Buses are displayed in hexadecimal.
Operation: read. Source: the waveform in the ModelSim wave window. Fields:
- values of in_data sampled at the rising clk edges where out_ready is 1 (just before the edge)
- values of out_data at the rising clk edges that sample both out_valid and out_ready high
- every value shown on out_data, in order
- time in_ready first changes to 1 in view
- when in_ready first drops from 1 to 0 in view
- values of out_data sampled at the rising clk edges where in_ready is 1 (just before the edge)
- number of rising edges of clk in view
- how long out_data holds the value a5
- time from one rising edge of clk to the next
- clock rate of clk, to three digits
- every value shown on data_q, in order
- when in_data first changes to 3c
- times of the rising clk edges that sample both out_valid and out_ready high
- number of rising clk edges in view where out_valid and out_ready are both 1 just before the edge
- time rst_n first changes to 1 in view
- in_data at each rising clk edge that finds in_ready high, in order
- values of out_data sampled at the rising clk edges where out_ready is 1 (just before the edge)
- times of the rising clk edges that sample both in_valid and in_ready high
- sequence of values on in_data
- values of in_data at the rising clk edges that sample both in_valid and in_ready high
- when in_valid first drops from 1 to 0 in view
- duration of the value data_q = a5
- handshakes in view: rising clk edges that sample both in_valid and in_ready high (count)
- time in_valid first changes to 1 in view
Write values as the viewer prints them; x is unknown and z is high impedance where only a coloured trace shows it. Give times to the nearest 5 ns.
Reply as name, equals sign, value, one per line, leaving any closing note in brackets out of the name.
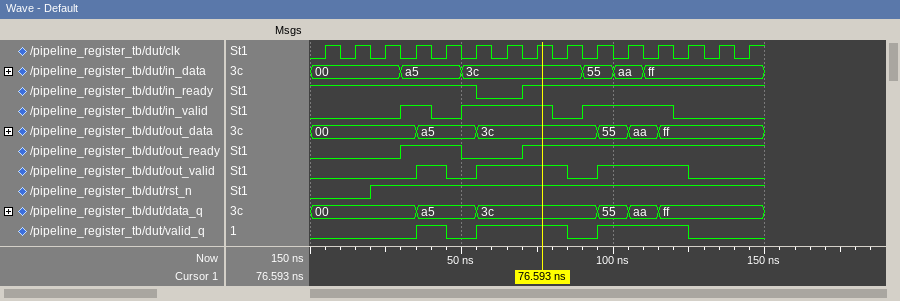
values of in_data sampled at the rising clk edges where out_ready is 1 = a5, a5, 3c, 3c, 55, aa, ff, ff, ff, ff
values of out_data at the rising clk edges that sample both out_valid and out_ready high = a5, 3c, 3c, 55, aa, ff
every value shown on out_data, in order = 00, a5, 3c, 55, aa, ff
time in_ready first changes to 1 in view = 70 ns
when in_ready first drops from 1 to 0 in view = 55 ns
values of out_data sampled at the rising clk edges where in_ready is 1 = 00, 00, 00, 00, a5, a5, 3c, 3c, 3c, 55, aa, ff, ff, ff
number of rising edges of clk in view = 15
how long out_data holds the value a5 = 20 ns
time from one rising edge of clk to the next = 10 ns
clock rate of clk, to three digits = 100 MHz
every value shown on data_q, in order = 00, a5, 3c, 55, aa, ff
when in_data first changes to 3c = 50 ns
times of the rising clk edges that sample both out_valid and out_ready high = 45 ns, 75 ns, 85 ns, 105 ns, 115 ns, 125 ns
number of rising clk edges in view where out_valid and out_ready are both 1 just before the edge = 6
time rst_n first changes to 1 in view = 20 ns
in_data at each rising clk edge that finds in_ready high, in order = 00, 00, 00, a5, a5, 3c, 3c, 3c, 55, aa, ff, ff, ff, ff
values of out_data sampled at the rising clk edges where out_ready is 1 = 00, a5, 3c, 3c, 3c, 55, aa, ff, ff, ff
times of the rising clk edges that sample both in_valid and in_ready high = 35 ns, 55 ns, 75 ns, 95 ns, 105 ns, 115 ns
sequence of values on in_data = 00, a5, 3c, 55, aa, ff
values of in_data at the rising clk edges that sample both in_valid and in_ready high = a5, 3c, 3c, 55, aa, ff
when in_valid first drops from 1 to 0 in view = 40 ns
duration of the value data_q = a5 = 20 ns
handshakes in view: rising clk edges that sample both in_valid and in_ready high = 6
time in_valid first changes to 1 in view = 30 ns
